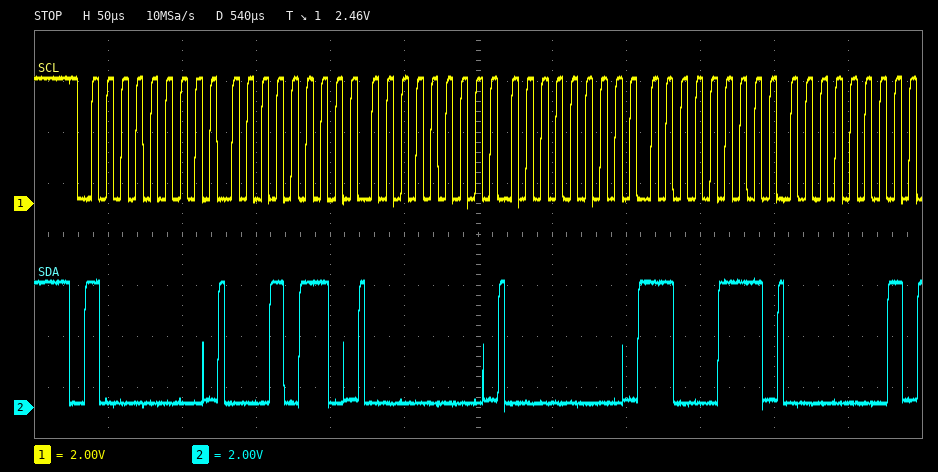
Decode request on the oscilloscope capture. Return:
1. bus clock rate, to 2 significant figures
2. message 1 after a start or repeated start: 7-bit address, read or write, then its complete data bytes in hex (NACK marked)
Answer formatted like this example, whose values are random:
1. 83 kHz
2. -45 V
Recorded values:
1. 100 kHz
2. 0x40 write: 16 00 00 C7 01
